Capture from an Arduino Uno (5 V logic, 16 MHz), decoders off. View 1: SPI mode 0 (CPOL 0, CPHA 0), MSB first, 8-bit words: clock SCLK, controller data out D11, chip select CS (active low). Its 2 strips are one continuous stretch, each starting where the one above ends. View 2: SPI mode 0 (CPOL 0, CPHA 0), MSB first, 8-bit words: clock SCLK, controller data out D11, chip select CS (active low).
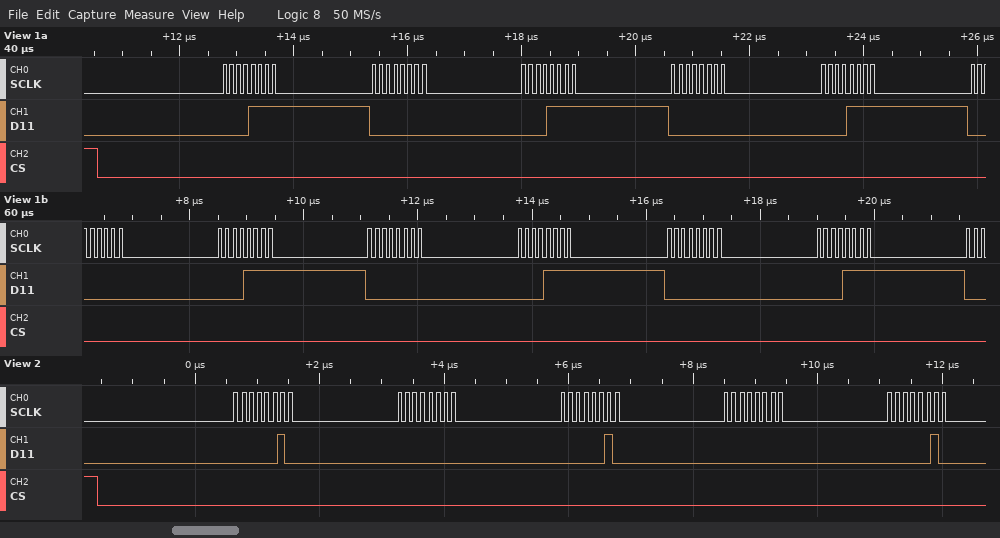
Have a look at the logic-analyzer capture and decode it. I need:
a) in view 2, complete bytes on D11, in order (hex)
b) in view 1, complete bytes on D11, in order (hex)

0x02 0x00 0x02 0x00 0x02
0F 00 0F 00 0F 00 0F 00 0F 00 0F
